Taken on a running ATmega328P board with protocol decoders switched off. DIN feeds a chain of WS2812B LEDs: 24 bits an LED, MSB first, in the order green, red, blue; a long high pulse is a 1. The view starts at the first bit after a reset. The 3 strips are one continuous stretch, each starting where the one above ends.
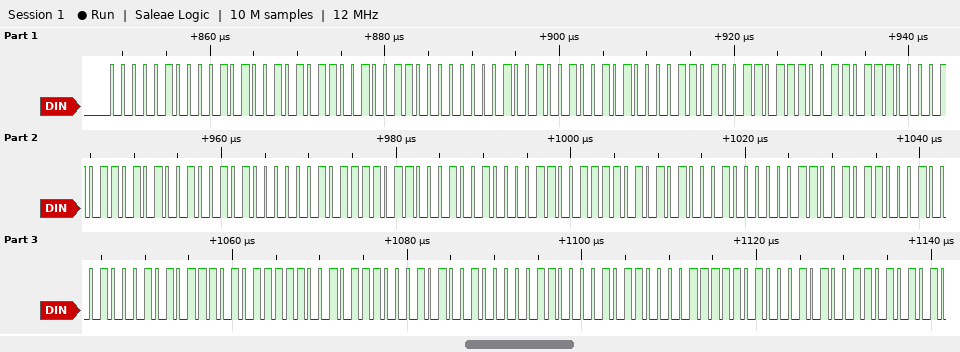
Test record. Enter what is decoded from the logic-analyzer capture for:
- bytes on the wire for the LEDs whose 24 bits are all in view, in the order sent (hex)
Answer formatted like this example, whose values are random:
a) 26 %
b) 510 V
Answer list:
a) 04 29 59 30 09 25 0D 37 37 0B 52 50 2F 62 43 3D 51 03 2C 44 57 5F 2E 29 06 16 1F
